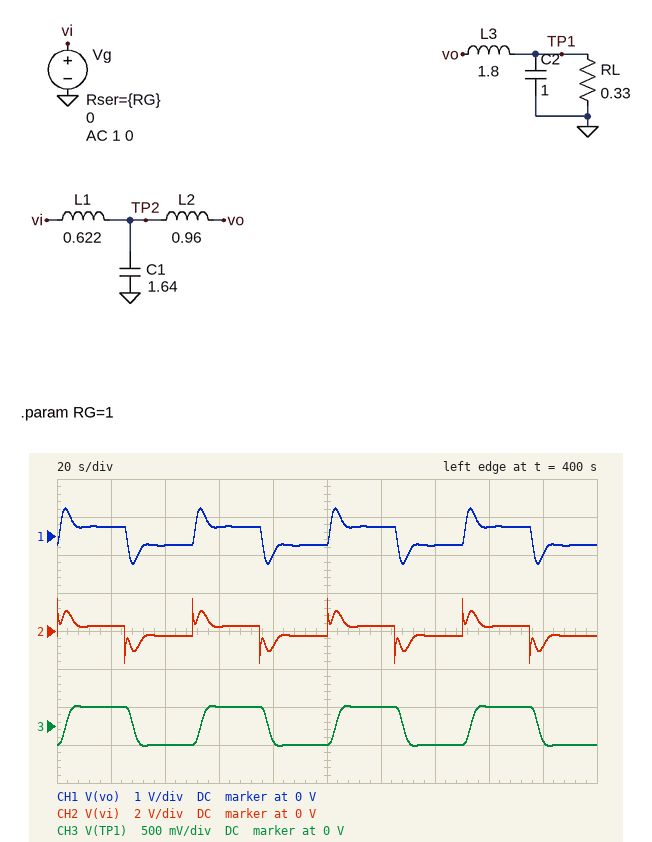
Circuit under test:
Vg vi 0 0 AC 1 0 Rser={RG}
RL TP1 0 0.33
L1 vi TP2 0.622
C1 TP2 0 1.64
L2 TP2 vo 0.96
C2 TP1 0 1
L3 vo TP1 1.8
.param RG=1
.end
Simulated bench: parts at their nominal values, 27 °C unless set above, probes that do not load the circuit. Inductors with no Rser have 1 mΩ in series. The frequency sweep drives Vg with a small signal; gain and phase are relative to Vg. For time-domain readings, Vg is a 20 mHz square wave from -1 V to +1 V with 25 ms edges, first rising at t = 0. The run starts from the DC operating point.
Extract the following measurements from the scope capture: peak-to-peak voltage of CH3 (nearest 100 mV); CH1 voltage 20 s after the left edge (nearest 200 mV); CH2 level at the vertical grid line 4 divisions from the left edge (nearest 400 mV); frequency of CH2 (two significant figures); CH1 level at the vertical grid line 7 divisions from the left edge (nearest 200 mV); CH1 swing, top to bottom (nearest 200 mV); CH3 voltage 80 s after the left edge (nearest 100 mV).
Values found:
500 mV
200 mV
-800 mV
20 mHz
-200 mV
1.4 V
-200 mV
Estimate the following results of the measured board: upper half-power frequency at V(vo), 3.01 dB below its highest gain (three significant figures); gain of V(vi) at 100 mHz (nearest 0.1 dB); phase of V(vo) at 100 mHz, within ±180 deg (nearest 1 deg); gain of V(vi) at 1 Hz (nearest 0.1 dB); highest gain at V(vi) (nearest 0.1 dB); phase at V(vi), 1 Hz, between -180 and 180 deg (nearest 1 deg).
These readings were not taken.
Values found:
173 mHz
-2.2 dB
-34 deg
-0.3 dB
0 dB
15 deg
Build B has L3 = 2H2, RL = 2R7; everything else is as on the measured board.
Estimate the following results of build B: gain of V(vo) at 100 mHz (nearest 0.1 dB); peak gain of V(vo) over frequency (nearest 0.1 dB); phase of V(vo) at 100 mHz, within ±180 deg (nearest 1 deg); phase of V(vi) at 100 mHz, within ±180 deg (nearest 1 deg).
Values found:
-7.4 dB
-2.7 dB
-54 deg
-5 deg
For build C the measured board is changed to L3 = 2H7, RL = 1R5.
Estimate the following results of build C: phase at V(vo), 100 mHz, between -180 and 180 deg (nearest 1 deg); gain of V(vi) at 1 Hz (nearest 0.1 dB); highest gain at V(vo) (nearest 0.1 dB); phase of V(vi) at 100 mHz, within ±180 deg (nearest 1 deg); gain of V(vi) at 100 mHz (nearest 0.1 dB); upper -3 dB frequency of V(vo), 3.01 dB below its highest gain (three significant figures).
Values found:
-43 deg
-0.3 dB
-4.4 dB
-23 deg
-3.7 dB
183 mHz
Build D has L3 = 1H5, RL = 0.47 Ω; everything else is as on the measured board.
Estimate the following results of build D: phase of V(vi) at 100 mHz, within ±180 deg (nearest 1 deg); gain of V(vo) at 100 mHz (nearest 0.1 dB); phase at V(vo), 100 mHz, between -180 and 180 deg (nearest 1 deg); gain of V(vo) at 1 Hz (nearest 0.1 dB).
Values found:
-19 deg
-5.3 dB
-35 deg
-36.5 dB
